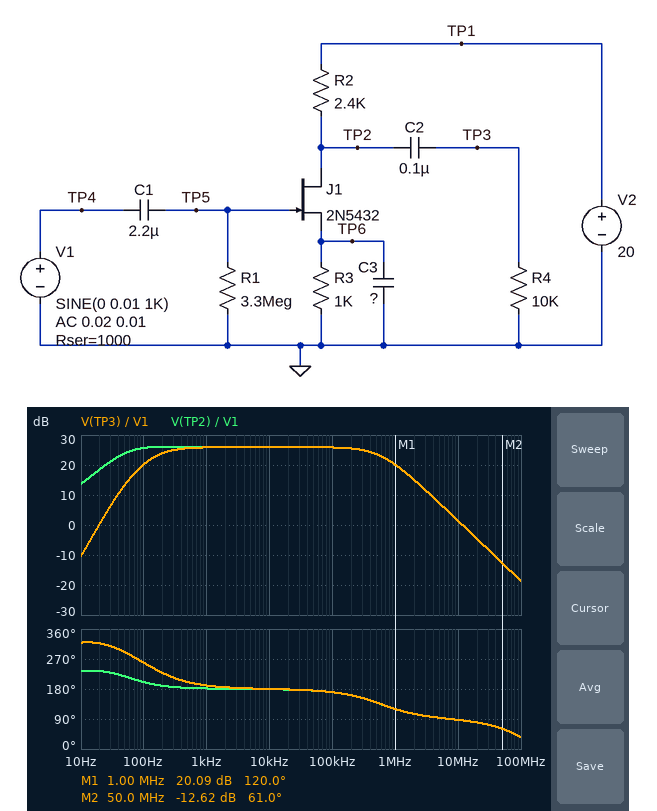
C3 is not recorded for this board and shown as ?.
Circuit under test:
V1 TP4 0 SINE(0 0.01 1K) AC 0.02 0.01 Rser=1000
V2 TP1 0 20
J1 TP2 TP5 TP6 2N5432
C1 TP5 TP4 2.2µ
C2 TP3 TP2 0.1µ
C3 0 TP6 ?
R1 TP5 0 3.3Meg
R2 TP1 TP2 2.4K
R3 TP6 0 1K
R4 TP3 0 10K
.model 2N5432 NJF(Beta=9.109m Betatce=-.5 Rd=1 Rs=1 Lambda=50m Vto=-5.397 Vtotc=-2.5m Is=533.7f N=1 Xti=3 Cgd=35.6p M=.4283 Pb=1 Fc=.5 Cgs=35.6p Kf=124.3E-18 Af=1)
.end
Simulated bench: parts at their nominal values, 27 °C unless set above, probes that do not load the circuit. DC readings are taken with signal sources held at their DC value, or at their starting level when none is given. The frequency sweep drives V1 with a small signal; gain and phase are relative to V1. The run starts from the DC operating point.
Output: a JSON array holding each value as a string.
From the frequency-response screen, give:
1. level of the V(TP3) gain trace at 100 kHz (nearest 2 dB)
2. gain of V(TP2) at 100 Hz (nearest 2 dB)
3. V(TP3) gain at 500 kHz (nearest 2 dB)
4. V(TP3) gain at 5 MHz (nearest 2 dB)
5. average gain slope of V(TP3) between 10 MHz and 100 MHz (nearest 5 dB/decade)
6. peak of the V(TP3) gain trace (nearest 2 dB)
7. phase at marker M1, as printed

["26 dB", "26 dB", "24 dB", "8 dB", "-20 dB/decade", "26 dB", "120.0 deg"]
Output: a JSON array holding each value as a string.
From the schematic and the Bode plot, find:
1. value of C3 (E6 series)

["33 µF"]
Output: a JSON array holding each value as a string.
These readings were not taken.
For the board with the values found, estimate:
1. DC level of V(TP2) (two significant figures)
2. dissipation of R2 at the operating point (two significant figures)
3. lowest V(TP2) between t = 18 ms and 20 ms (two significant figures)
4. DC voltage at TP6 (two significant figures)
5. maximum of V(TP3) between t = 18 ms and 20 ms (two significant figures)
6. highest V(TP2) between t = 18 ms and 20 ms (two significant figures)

["8.6 V", "54 mW", "8.4 V", "4.7 V", "200 mV", "8.8 V"]
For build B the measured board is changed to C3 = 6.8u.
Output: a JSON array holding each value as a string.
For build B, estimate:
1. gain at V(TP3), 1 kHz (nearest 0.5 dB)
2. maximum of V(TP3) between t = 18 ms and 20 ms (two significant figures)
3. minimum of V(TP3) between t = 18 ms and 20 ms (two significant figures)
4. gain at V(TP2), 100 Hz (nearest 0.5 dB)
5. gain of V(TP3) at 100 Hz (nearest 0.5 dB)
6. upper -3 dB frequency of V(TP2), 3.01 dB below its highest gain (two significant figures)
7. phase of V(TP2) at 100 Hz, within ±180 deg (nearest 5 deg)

["25.5 dB", "190 mV", "-190 mV", "18.0 dB", "12.5 dB", "590 kHz", "-130 deg"]
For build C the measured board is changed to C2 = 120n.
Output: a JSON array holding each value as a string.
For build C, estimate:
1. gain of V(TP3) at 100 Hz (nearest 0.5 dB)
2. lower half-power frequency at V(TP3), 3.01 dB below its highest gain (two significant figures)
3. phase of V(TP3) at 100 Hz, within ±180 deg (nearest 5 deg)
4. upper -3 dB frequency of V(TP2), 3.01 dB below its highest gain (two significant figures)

["21.0 dB", "140 Hz", "-105 deg", "590 kHz"]
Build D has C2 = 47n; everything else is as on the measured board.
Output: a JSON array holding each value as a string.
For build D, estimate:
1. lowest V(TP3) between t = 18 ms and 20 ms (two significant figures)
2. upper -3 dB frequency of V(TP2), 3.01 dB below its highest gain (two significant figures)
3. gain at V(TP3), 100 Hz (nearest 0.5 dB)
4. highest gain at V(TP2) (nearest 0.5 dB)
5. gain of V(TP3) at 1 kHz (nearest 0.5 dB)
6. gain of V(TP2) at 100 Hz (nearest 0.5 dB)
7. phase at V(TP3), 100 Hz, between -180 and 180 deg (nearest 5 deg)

["-190 mV", "510 kHz", "15.0 dB", "26.5 dB", "25.5 dB", "26.0 dB", "-85 deg"]
